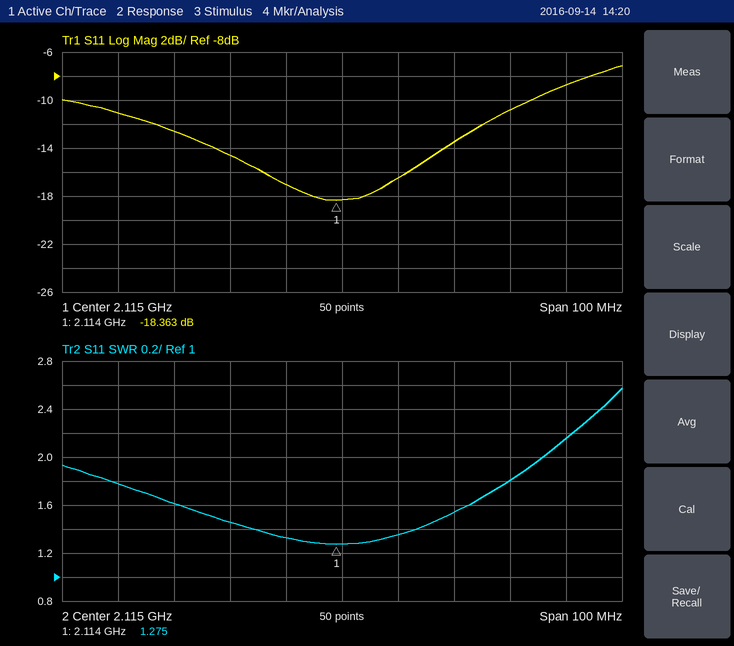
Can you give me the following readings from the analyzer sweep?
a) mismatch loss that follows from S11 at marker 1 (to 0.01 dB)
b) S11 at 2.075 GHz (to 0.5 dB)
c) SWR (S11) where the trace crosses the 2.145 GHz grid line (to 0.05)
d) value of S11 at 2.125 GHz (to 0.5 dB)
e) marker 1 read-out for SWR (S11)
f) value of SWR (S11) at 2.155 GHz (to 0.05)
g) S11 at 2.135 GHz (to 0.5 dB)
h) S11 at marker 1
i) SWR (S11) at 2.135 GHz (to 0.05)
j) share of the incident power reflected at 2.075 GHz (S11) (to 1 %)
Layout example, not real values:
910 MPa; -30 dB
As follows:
0.06 dB; -11.0 dB; 1.80; -16.5 dB; 1.275; 2.15; -13.5 dB; -18.363 dB; 1.55; 8 %
